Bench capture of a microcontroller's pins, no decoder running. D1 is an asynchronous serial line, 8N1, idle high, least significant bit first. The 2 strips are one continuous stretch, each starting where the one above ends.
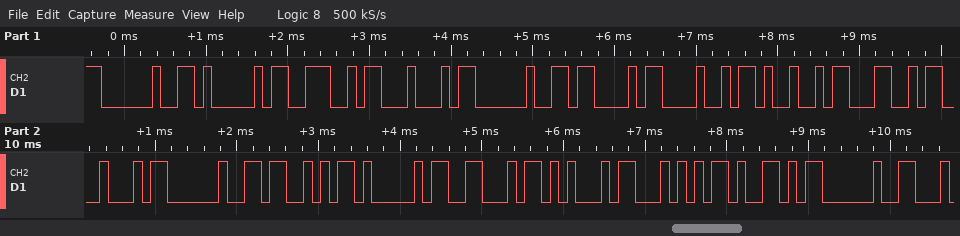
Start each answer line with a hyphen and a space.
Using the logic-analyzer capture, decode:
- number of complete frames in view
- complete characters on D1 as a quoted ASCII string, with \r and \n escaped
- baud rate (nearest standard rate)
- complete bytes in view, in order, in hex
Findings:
- 18
- " AND CHILD SAFETY "
- 9600 baud
- 20 41 4E 44 20 43 48 49 4C 44 20 53 41 46 45 54 59 20
